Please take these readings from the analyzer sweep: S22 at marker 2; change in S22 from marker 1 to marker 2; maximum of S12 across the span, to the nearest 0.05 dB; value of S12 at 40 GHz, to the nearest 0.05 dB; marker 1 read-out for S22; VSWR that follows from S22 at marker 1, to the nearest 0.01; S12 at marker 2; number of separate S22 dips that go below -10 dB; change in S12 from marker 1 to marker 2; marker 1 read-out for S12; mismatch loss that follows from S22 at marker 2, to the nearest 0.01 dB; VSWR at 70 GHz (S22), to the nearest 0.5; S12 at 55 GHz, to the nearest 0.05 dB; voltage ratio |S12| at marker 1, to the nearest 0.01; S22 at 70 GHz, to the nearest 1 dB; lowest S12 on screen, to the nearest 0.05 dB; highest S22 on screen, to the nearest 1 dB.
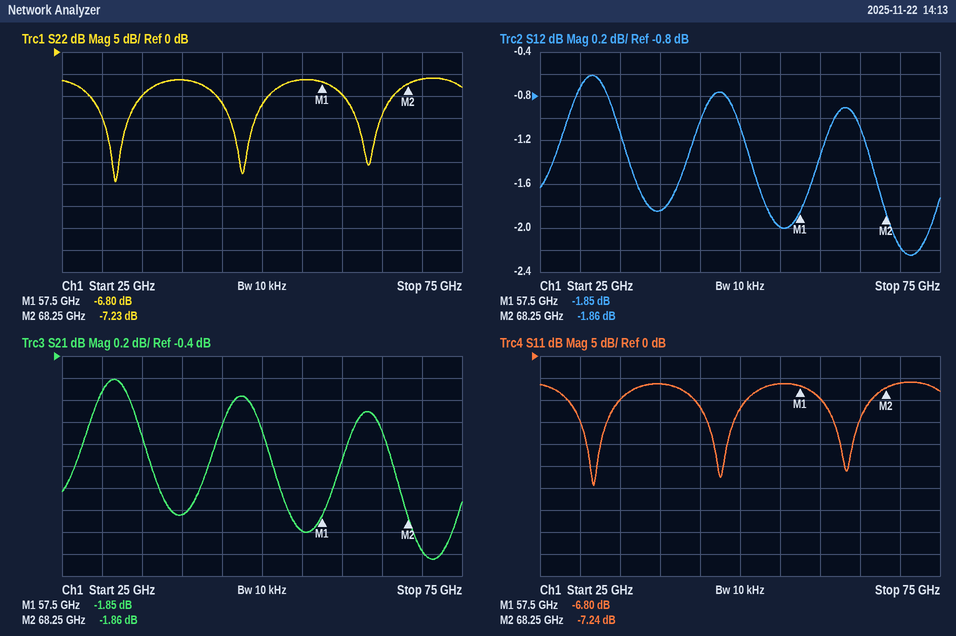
-7.23 dB
-0.43 dB
-0.60 dB
-1.85 dB
-6.80 dB
2.68
-1.86 dB
3
-0.01 dB
-1.85 dB
0.91 dB
3.0
-2.00 dB
0.81
-6 dB
-2.25 dB
-6 dB
